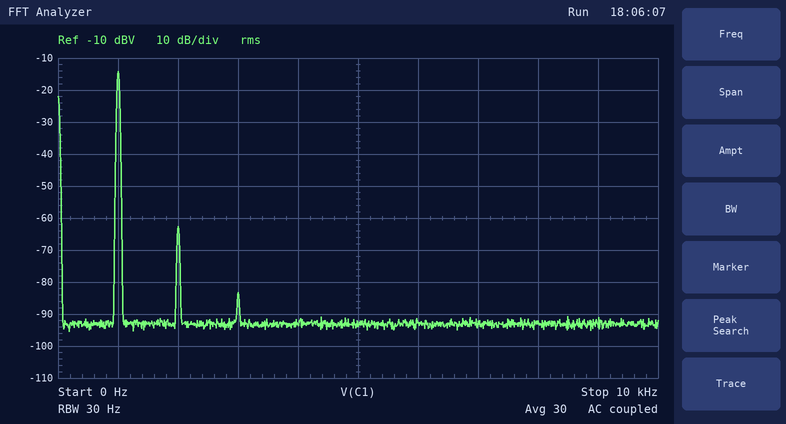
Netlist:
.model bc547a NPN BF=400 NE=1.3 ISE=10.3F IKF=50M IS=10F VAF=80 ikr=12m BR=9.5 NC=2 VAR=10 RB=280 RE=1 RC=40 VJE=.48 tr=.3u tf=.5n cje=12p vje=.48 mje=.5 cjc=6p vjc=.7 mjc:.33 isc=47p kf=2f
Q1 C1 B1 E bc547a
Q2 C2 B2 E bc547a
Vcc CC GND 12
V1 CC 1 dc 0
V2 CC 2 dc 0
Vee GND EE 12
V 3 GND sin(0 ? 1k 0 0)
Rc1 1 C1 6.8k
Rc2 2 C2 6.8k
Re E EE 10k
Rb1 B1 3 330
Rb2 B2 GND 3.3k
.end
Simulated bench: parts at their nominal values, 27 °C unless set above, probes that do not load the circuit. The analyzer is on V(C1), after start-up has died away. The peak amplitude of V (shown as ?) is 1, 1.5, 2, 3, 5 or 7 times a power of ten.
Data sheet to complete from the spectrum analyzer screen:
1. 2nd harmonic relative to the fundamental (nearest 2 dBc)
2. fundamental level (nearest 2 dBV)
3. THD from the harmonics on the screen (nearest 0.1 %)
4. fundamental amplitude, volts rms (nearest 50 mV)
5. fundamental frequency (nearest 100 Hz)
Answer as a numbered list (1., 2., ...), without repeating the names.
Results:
1. -48 dBc
2. -14 dBV
3. 0.4 %
4. 200 mV
5. 1.0 kHz
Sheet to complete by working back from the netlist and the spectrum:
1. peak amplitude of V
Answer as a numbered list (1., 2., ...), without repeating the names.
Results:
1. 5 mV
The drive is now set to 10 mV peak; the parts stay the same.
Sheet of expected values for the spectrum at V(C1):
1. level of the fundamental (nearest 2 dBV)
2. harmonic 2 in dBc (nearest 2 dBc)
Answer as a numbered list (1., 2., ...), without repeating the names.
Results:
1. -8 dBV
2. -42 dBc
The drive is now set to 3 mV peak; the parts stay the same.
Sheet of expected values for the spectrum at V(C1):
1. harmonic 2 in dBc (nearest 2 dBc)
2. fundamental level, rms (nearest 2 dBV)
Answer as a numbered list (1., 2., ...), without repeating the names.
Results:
1. -52 dBc
2. -18 dBV
